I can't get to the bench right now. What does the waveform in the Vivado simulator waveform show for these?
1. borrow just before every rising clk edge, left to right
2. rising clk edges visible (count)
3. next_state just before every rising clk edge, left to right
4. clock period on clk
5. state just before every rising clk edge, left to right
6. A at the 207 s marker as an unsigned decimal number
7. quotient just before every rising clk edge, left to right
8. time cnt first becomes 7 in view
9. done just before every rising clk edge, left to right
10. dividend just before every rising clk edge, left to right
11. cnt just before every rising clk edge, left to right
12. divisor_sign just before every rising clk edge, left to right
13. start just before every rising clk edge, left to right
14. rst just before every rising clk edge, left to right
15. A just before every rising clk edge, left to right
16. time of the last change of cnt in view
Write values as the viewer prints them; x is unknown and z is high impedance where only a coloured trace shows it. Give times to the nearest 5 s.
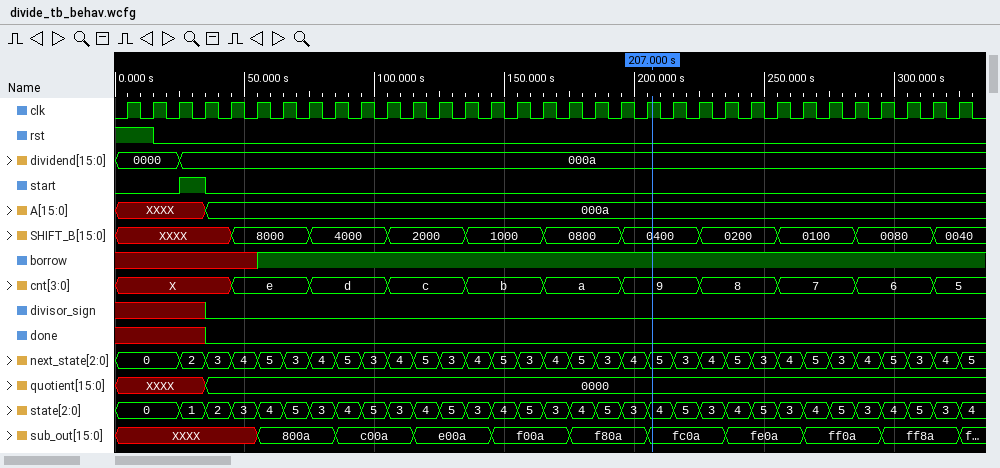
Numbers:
x x x x x x 1 1 1 1 1 1 1 1 1 1 1 1 1 1 1 1 1 1 1 1 1 1 1 1 1 1 1
33
0, 0, 0, 2, 3, 4, 5, 3, 4, 5, 3, 4, 5, 3, 4, 5, 3, 4, 5, 3, 4, 5, 3, 4, 5, 3, 4, 5, 3, 4, 5, 3, 4
10 s
0, 0, 0, 1, 2, 3, 4, 5, 3, 4, 5, 3, 4, 5, 3, 4, 5, 3, 4, 5, 3, 4, 5, 3, 4, 5, 3, 4, 5, 3, 4, 5, 3
10
XXXX, XXXX, XXXX, XXXX, 0000, 0000, 0000, 0000, 0000, 0000, 0000, 0000, 0000, 0000, 0000, 0000, 0000, 0000, 0000, 0000, 0000, 0000, 0000, 0000, 0000, 0000, 0000, 0000, 0000, 0000, 0000, 0000, 0000
255 s
x x x x 0 0 0 0 0 0 0 0 0 0 0 0 0 0 0 0 0 0 0 0 0 0 0 0 0 0 0 0 0
0000, 0000, 0000, 000a, 000a, 000a, 000a, 000a, 000a, 000a, 000a, 000a, 000a, 000a, 000a, 000a, 000a, 000a, 000a, 000a, 000a, 000a, 000a, 000a, 000a, 000a, 000a, 000a, 000a, 000a, 000a, 000a, 000a
X, X, X, X, X, e, e, e, d, d, d, c, c, c, b, b, b, a, a, a, 9, 9, 9, 8, 8, 8, 7, 7, 7, 6, 6, 6, 5
x x x x 0 0 0 0 0 0 0 0 0 0 0 0 0 0 0 0 0 0 0 0 0 0 0 0 0 0 0 0 0
0 0 0 1 0 0 0 0 0 0 0 0 0 0 0 0 0 0 0 0 0 0 0 0 0 0 0 0 0 0 0 0 0
1 1 0 0 0 0 0 0 0 0 0 0 0 0 0 0 0 0 0 0 0 0 0 0 0 0 0 0 0 0 0 0 0
XXXX, XXXX, XXXX, XXXX, 000a, 000a, 000a, 000a, 000a, 000a, 000a, 000a, 000a, 000a, 000a, 000a, 000a, 000a, 000a, 000a, 000a, 000a, 000a, 000a, 000a, 000a, 000a, 000a, 000a, 000a, 000a, 000a, 000a
315 s
